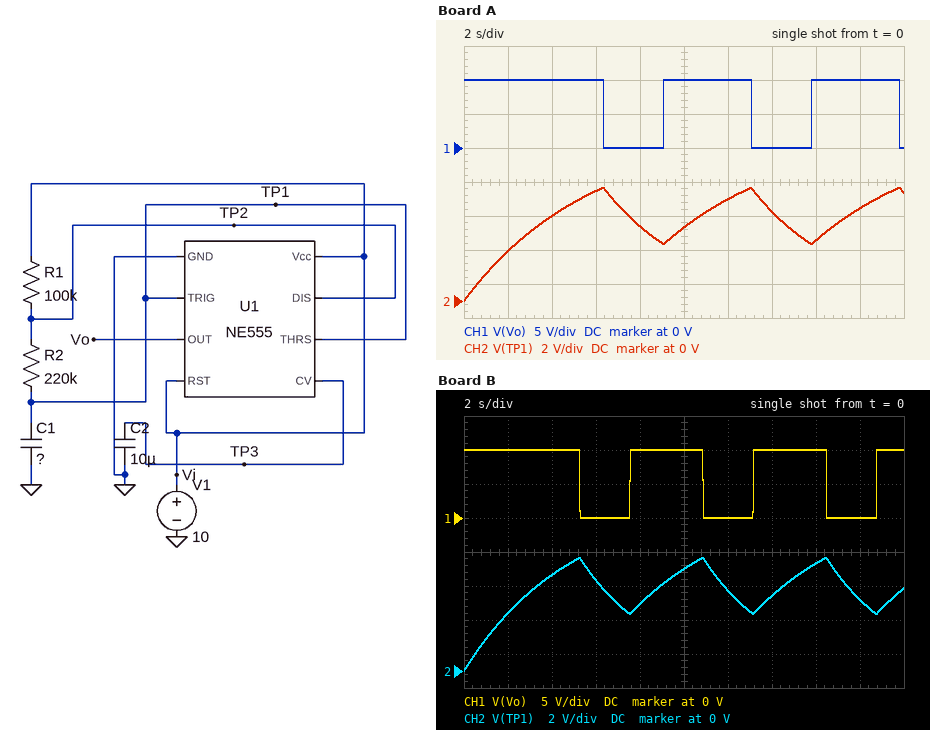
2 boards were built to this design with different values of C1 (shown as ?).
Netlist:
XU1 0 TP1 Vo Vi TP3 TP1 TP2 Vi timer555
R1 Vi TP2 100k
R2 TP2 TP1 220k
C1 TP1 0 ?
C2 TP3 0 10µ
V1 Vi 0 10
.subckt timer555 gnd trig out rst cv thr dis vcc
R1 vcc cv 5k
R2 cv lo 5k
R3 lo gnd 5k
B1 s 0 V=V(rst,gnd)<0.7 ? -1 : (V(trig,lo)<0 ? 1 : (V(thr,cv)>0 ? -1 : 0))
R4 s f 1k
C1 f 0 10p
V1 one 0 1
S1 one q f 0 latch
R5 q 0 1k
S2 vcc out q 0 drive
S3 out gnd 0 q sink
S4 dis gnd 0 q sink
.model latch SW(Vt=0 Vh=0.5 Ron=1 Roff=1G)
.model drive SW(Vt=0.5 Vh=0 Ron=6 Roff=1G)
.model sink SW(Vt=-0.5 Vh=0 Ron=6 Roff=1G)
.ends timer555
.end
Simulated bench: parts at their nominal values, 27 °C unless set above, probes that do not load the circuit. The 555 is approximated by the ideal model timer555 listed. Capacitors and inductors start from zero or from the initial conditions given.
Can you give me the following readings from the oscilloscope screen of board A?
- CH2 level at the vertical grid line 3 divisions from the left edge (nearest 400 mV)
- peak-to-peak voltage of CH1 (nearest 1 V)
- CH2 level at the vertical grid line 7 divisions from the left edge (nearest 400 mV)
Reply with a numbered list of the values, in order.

1. 6.4 V
2. 10 V
3. 5.2 V
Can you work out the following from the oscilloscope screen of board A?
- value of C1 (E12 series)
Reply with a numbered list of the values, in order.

1. 18 µF
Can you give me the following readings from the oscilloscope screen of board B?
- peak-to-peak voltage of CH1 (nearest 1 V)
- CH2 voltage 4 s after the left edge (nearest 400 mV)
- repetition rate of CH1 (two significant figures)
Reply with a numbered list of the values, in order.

1. 10 V
2. 5.6 V
3. 180 mHz
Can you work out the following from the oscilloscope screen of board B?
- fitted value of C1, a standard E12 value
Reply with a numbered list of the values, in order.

1. 15 µF
